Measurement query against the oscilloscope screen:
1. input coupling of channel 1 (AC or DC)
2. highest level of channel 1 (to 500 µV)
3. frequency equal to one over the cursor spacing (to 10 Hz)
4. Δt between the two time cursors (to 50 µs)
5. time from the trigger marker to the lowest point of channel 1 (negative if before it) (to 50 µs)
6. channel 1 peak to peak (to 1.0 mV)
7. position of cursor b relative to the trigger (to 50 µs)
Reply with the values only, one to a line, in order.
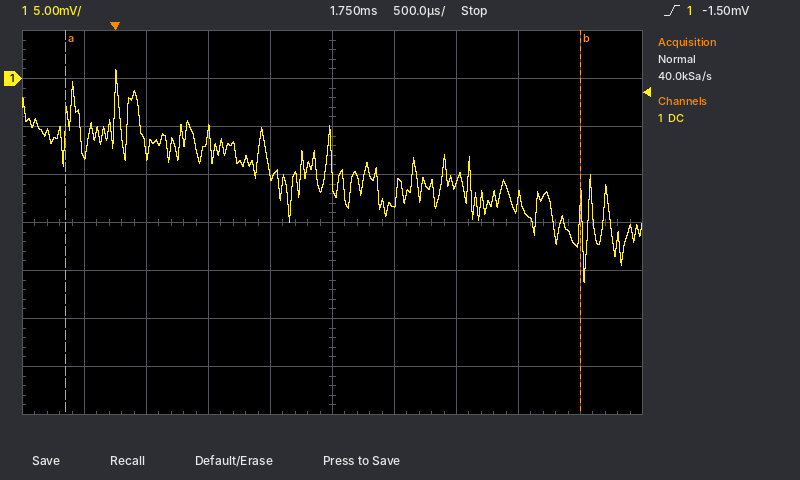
DC
1.0 mV
240 Hz
4.15 ms
+3.80 ms
22.0 mV
+3.75 ms
